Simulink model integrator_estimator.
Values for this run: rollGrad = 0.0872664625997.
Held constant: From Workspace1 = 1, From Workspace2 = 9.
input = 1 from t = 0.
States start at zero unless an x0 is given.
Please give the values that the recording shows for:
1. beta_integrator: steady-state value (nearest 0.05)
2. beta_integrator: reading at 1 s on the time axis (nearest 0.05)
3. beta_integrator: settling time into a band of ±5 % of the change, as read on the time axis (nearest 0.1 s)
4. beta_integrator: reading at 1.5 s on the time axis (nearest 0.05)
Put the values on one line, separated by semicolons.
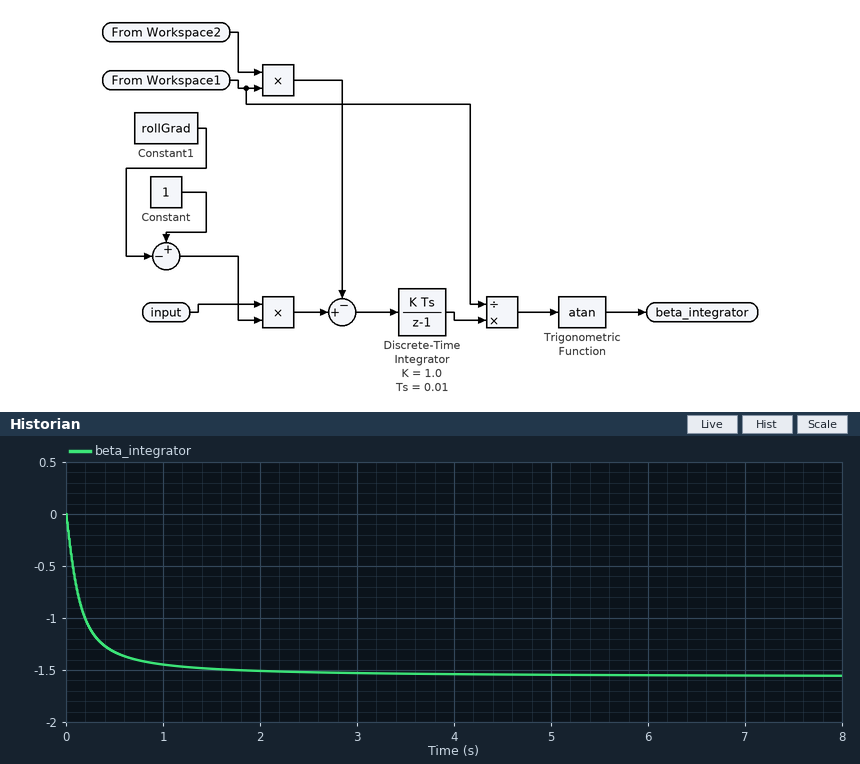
-1.55; -1.45; 1.5 s; -1.50
